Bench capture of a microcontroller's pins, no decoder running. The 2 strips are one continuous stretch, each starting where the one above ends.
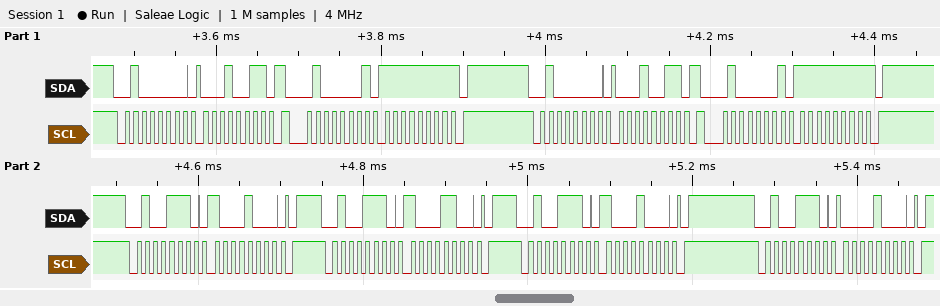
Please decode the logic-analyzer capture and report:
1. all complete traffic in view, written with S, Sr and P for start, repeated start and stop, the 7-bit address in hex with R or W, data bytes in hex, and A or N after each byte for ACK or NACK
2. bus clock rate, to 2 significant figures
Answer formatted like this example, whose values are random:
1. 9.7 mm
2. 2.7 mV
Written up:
1. S 20W A 13 A Sr 20R A FF N P S 20W A 13 A Sr 20R A FF N P S 27W A 88 A P S 27W A 8C A P S 27W A 88 A P S 27W A 08 A P
2. 100 kHz
